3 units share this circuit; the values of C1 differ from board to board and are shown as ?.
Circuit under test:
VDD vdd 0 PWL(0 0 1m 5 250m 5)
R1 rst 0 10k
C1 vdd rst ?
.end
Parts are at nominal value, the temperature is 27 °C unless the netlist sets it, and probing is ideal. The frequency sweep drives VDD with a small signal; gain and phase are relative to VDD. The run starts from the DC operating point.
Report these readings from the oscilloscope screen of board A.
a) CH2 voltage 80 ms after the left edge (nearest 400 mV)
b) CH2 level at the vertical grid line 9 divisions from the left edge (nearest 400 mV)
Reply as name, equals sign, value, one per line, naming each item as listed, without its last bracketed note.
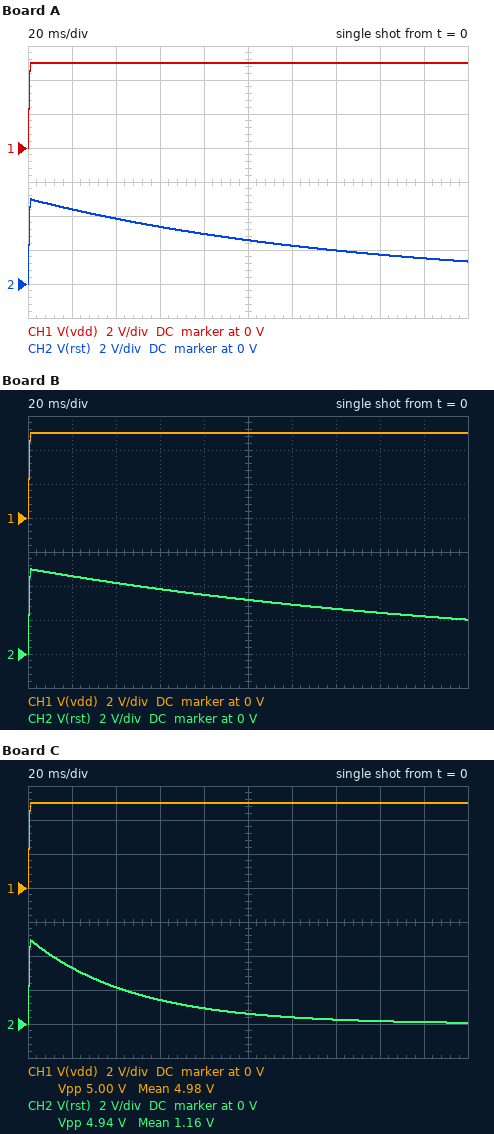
CH2 voltage 80 ms after the left edge = 2.8 V
CH2 level at the vertical grid line 9 divisions from the left edge = 1.6 V
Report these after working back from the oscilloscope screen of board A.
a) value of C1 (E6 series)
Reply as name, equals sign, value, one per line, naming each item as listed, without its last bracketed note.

value of C1 = 15 µF
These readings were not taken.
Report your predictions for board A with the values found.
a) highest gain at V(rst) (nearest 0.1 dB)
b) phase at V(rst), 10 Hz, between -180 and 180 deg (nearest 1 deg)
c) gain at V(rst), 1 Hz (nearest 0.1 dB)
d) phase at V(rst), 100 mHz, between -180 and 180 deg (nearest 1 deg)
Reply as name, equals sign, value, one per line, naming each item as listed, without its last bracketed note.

highest gain at V(rst) = 0 dB
phase at V(rst), 10 Hz, between -180 and 180 deg = 6 deg
gain at V(rst), 1 Hz = -3.3 dB
phase at V(rst), 100 mHz, between -180 and 180 deg = 85 deg
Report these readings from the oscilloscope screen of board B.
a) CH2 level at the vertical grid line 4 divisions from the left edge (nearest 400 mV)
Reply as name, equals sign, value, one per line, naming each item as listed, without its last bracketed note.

CH2 level at the vertical grid line 4 divisions from the left edge = 3.6 V
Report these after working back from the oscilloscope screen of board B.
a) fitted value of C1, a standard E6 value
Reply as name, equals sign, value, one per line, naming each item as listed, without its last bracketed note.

fitted value of C1, a standard E6 value = 22 µF
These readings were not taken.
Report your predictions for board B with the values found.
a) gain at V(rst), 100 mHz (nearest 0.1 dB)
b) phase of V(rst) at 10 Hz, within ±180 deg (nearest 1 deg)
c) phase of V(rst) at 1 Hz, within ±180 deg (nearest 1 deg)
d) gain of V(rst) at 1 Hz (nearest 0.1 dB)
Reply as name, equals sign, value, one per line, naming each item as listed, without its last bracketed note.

gain at V(rst), 100 mHz = -17.3 dB
phase of V(rst) at 10 Hz, within ±180 deg = 4 deg
phase of V(rst) at 1 Hz, within ±180 deg = 36 deg
gain of V(rst) at 1 Hz = -1.8 dB
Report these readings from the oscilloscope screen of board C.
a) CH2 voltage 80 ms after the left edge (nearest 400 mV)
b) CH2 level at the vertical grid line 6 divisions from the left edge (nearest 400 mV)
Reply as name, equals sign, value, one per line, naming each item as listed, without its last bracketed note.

CH2 voltage 80 ms after the left edge = 800 mV
CH2 level at the vertical grid line 6 divisions from the left edge = 400 mV
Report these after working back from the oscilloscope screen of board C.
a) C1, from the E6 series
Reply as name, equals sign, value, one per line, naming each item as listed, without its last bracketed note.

C1, from the E6 series = 4.7 µF
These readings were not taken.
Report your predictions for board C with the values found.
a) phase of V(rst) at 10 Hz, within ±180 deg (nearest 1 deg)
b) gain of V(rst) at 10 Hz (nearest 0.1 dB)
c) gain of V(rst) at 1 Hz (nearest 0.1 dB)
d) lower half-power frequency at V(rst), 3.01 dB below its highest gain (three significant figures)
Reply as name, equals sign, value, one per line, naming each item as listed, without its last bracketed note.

phase of V(rst) at 10 Hz, within ±180 deg = 19 deg
gain of V(rst) at 10 Hz = -0.5 dB
gain of V(rst) at 1 Hz = -11.0 dB
lower half-power frequency at V(rst), 3.01 dB below its highest gain = 3.39 Hz
